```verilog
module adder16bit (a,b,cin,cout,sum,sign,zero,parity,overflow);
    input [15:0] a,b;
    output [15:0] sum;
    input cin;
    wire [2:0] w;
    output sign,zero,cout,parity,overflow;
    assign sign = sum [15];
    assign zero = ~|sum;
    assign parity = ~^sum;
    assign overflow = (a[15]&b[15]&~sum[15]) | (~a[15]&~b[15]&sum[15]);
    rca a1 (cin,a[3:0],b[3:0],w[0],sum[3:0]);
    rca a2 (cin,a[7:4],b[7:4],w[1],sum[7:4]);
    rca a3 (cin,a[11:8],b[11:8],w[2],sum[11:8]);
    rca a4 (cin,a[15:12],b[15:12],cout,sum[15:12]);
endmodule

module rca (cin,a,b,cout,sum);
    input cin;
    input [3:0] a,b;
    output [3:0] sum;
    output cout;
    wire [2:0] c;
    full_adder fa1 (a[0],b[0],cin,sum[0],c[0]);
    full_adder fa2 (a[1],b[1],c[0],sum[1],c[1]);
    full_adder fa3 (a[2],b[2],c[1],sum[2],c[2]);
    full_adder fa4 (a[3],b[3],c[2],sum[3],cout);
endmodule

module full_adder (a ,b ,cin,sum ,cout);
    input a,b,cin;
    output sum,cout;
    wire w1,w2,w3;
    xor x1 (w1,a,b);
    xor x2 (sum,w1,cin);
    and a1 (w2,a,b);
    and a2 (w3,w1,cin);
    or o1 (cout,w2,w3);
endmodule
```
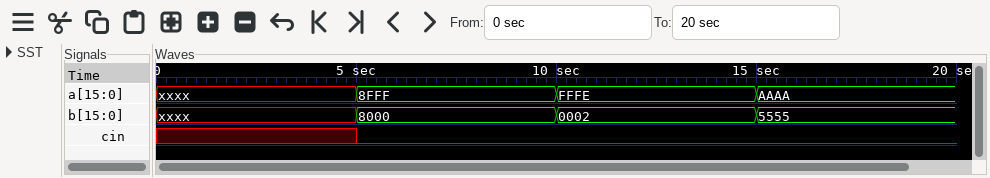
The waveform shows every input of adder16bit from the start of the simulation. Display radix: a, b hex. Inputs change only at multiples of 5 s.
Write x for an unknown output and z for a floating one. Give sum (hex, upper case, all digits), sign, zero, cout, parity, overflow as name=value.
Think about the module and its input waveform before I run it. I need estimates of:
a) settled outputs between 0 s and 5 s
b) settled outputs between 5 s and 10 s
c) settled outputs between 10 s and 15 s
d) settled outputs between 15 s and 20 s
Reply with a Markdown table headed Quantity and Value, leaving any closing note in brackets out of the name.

| Quantity | Value |
|---|---|
| settled outputs between 0 s and 5 s | sum=x, sign=x, zero=x, cout=x, parity=x, overflow=x |
| settled outputs between 5 s and 10 s | sum=0FFF, sign=0, zero=0, cout=1, parity=1, overflow=1 |
| settled outputs between 10 s and 15 s | sum=FFF0, sign=1, zero=0, cout=0, parity=1, overflow=0 |
| settled outputs between 15 s and 20 s | sum=FFFF, sign=1, zero=0, cout=0, parity=1, overflow=0 |
